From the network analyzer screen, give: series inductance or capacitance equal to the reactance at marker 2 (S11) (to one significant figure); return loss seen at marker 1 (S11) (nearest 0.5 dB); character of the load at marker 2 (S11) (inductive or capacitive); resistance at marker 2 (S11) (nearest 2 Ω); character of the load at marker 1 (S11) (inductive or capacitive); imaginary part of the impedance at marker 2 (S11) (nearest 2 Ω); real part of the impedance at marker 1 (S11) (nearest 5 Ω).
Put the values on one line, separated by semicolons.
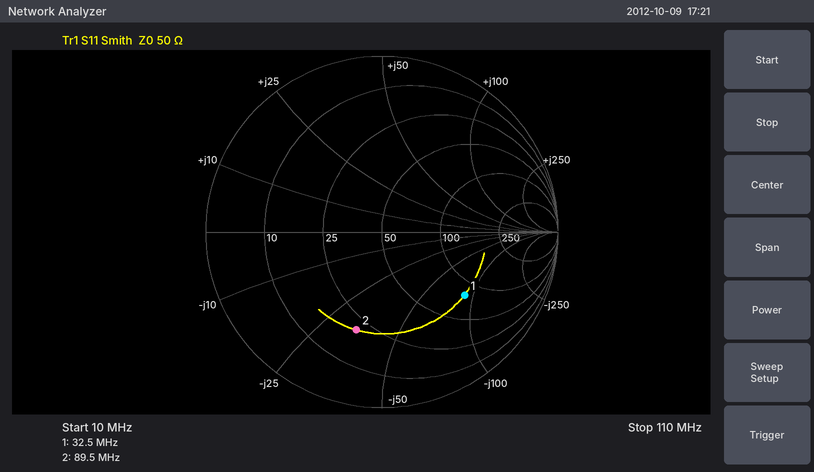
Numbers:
50 pF; 4.5 dB; capacitive; 20 Ω; capacitive; -34 Ω; 80 Ω
